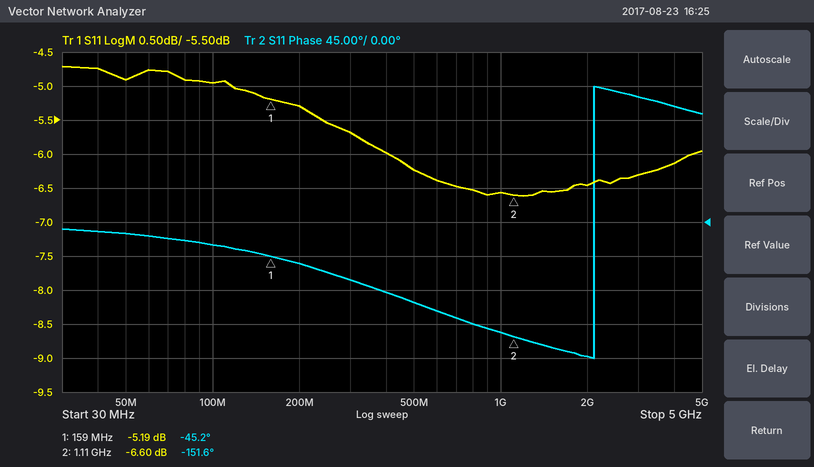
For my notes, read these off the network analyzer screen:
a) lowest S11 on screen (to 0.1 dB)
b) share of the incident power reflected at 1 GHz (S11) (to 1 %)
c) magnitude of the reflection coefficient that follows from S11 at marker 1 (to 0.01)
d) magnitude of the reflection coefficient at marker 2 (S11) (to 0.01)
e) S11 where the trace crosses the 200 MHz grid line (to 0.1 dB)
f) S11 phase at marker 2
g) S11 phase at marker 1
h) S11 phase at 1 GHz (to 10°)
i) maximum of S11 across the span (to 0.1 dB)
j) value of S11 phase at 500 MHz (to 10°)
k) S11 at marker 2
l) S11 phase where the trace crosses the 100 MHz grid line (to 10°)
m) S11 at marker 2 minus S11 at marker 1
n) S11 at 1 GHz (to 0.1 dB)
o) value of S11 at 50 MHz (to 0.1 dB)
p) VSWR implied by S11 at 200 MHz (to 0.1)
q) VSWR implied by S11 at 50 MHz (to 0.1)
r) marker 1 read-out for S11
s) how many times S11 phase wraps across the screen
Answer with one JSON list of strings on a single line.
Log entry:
["-6.6 dB", "22 %", "0.55", "0.47", "-5.3 dB", "-151.6°", "-45.2°", "-150°", "-4.7 dB", "-110°", "-6.60 dB", "-30°", "-1.41 dB", "-6.6 dB", "-4.9 dB", "3.4", "3.6", "-5.19 dB", "1"]
